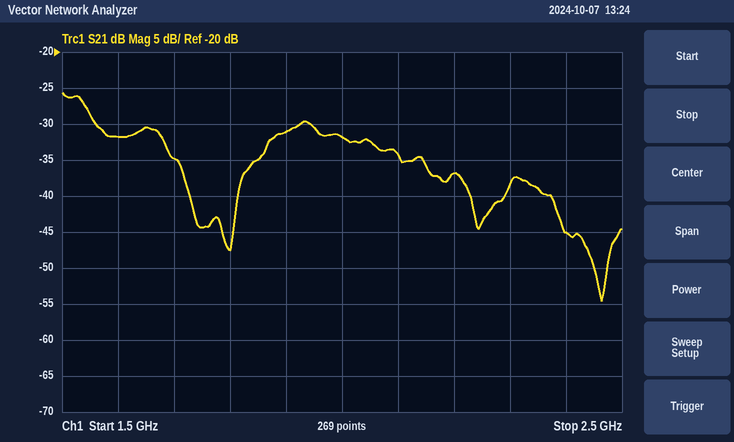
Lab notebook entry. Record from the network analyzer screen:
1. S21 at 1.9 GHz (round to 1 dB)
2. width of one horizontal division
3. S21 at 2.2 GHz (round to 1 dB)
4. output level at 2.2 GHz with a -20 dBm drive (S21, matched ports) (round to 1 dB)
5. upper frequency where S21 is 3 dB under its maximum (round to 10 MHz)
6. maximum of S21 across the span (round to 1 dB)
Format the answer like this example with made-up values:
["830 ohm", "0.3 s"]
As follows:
["-31 dB", "100 MHz", "-37 dB", "-57 dBm", "1.55 GHz", "-26 dB"]
